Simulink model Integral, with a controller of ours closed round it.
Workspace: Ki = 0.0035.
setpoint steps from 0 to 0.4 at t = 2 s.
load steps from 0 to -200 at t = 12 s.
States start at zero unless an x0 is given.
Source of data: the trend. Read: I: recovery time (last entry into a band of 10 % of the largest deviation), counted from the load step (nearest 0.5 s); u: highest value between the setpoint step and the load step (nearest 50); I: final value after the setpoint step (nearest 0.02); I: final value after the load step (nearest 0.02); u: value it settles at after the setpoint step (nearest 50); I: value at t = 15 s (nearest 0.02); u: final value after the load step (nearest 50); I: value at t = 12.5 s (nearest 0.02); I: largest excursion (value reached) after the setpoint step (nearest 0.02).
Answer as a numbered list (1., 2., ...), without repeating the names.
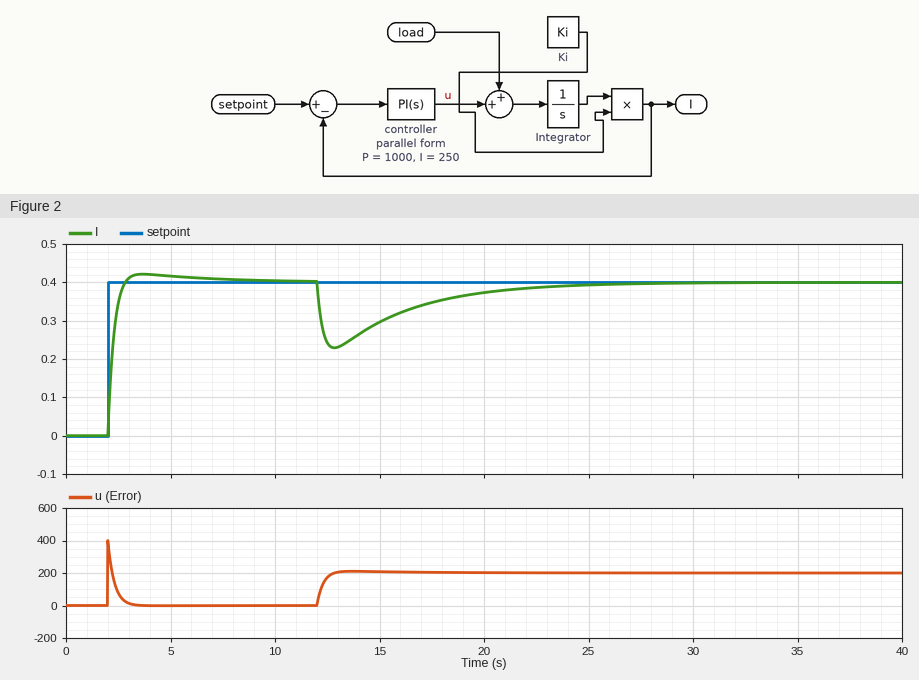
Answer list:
1. 9.5 s
2. 400
3. 0.40
4. 0.40
5. 0
6. 0.30
7. 200
8. 0.24
9. 0.42
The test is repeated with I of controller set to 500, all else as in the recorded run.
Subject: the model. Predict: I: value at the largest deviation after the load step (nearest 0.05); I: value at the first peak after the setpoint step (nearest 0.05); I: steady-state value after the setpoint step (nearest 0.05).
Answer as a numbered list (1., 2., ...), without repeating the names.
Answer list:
1. 0.25
2. 0.45
3. 0.40
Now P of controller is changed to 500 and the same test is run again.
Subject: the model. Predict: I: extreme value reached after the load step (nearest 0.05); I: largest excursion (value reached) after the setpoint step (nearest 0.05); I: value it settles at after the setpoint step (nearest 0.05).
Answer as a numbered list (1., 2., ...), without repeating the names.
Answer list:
1. 0.10
2. 0.45
3. 0.40
